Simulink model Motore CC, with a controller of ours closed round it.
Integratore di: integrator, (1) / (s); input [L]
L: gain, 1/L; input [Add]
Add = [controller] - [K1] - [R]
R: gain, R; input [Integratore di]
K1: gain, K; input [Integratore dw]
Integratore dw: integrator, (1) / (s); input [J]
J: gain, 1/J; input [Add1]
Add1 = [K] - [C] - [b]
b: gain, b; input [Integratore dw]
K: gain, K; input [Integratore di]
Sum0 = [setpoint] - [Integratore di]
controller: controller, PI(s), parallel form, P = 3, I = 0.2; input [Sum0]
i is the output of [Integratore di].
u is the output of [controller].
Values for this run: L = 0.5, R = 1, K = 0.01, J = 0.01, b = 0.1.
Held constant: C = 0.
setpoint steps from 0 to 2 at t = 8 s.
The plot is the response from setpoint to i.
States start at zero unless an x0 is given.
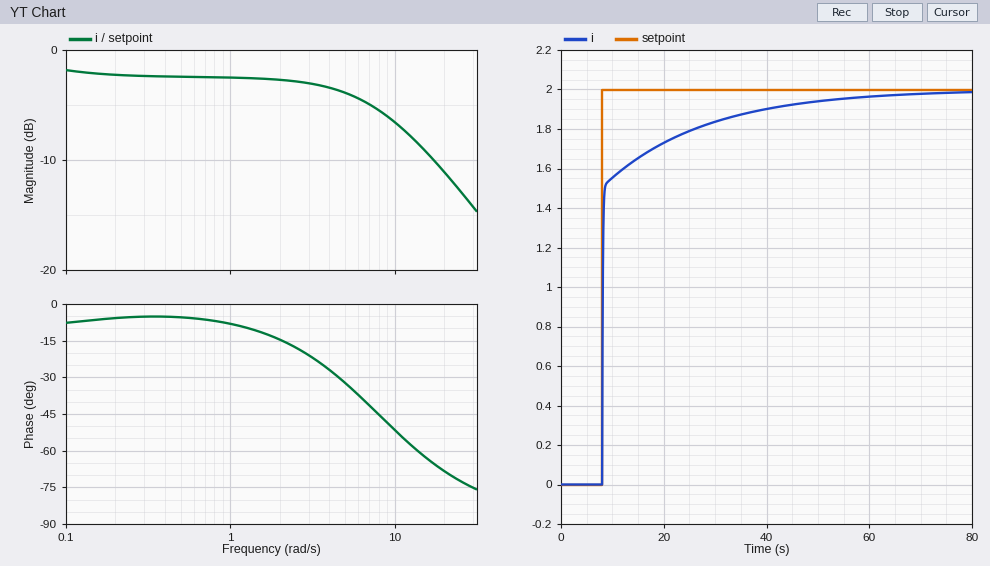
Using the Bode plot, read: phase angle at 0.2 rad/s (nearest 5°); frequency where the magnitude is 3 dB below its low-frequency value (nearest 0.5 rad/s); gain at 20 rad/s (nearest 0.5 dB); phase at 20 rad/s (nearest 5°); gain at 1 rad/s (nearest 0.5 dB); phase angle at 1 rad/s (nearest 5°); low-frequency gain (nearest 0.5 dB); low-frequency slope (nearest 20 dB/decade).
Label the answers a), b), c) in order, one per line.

a) -5°
b) 7.0 rad/s
c) -11.0 dB
d) -70°
e) -2.5 dB
f) -10°
g) -2.0 dB
h) 0 dB/decade
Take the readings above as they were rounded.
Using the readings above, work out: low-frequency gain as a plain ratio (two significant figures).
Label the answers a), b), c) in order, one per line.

a) 0.79
